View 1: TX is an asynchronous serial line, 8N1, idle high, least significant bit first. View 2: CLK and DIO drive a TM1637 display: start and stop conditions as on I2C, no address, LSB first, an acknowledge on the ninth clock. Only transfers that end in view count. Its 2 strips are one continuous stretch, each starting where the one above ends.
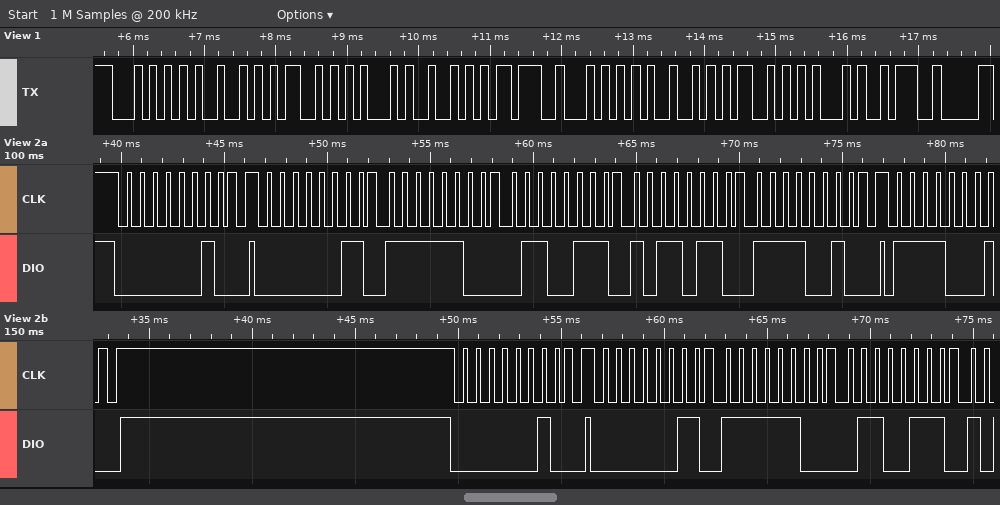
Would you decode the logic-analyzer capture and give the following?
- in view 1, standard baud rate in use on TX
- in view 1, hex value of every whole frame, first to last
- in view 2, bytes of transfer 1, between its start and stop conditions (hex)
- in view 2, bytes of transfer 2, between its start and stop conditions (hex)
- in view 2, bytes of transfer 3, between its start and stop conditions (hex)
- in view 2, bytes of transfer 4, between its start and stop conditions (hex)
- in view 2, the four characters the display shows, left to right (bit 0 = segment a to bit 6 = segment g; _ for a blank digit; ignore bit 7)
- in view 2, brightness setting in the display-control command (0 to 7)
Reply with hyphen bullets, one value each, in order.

- 9600 baud
- 54 49 4D 45 52 3B 54 49 4D 45 3A
- 40
- C0 3F E6 6D 4F
- 8F
- 40
- 0453
- 7
